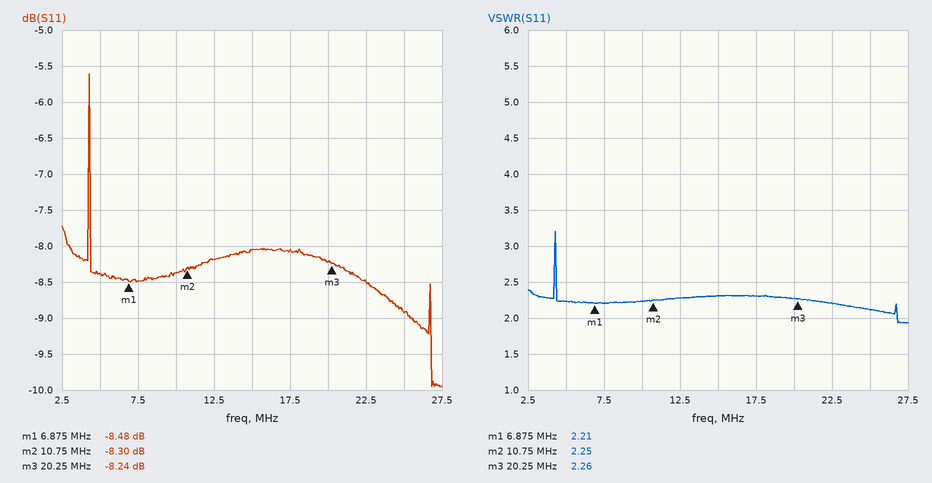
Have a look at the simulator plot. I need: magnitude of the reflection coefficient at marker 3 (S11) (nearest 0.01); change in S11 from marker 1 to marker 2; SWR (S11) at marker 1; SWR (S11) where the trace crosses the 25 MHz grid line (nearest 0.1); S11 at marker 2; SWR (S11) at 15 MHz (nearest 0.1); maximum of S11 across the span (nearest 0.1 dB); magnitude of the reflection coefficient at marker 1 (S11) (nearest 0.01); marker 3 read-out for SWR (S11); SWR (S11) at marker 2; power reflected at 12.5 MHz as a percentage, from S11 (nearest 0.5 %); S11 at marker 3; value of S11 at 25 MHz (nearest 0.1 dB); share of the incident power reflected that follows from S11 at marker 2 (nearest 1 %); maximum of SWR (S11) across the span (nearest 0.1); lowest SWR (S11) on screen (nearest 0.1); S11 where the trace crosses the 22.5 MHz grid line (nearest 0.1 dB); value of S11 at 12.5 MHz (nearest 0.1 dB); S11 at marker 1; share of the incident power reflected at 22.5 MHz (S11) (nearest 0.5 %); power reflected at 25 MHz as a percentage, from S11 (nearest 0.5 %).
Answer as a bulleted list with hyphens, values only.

- 0.39
- 0.18 dB
- 2.21
- 2.1
- -8.30 dB
- 2.3
- -5.6 dB
- 0.38
- 2.26
- 2.25
- 15.0 %
- -8.24 dB
- -8.9 dB
- 15 %
- 3.2
- 1.9
- -8.5 dB
- -8.2 dB
- -8.48 dB
- 14.0 %
- 13.0 %
